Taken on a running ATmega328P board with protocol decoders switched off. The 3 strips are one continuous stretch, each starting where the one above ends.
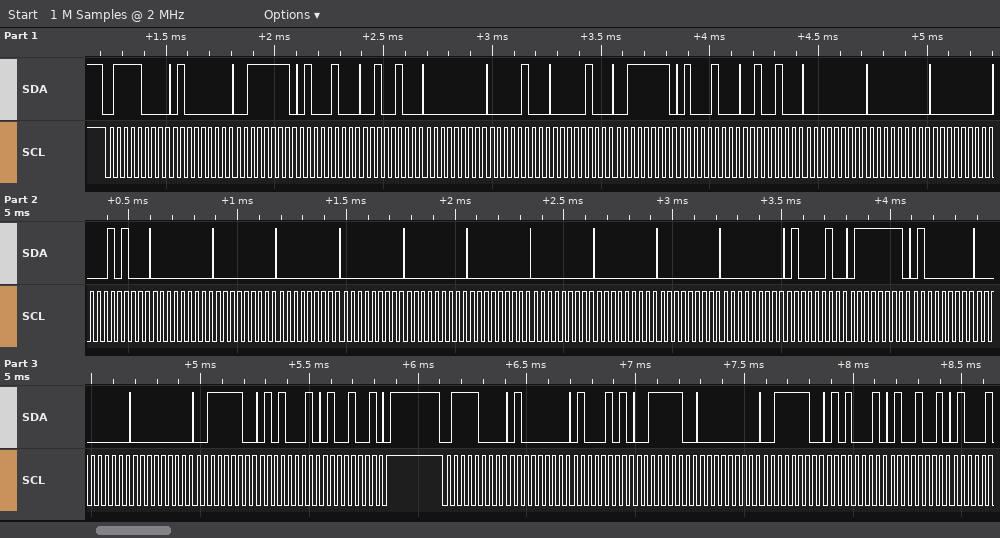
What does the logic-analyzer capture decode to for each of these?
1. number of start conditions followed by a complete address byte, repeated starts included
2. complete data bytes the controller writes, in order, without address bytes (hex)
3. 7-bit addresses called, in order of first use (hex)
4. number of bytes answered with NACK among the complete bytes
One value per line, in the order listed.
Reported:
2
40 3F 44 24 00 04 04 3F 44 24 00 00 00 14 00 00 00 00 00 00 00 00 00 00 42 7F 40 00 00 3E 51 49 40 45 3E 00 3E 51 49
0x3C
0
